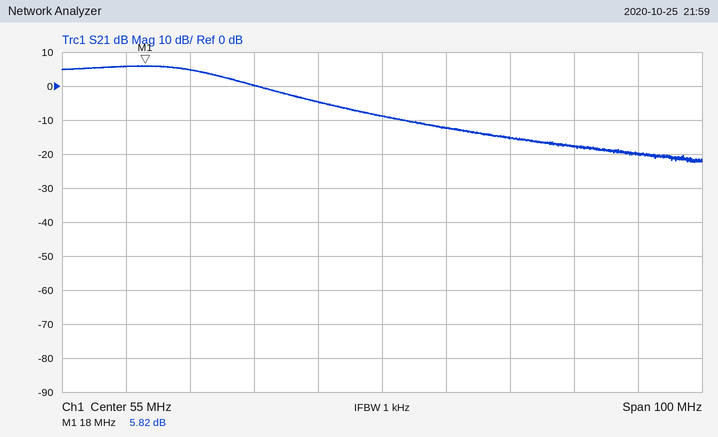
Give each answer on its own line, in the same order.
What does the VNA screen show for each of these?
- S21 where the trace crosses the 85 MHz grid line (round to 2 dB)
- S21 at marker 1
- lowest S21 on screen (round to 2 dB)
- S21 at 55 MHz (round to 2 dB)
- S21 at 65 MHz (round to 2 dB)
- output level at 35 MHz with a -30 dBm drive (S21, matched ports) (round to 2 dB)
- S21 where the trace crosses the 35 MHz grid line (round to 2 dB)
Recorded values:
-18 dB
5.82 dB
-22 dB
-8 dB
-12 dB
-30 dBm
0 dB
